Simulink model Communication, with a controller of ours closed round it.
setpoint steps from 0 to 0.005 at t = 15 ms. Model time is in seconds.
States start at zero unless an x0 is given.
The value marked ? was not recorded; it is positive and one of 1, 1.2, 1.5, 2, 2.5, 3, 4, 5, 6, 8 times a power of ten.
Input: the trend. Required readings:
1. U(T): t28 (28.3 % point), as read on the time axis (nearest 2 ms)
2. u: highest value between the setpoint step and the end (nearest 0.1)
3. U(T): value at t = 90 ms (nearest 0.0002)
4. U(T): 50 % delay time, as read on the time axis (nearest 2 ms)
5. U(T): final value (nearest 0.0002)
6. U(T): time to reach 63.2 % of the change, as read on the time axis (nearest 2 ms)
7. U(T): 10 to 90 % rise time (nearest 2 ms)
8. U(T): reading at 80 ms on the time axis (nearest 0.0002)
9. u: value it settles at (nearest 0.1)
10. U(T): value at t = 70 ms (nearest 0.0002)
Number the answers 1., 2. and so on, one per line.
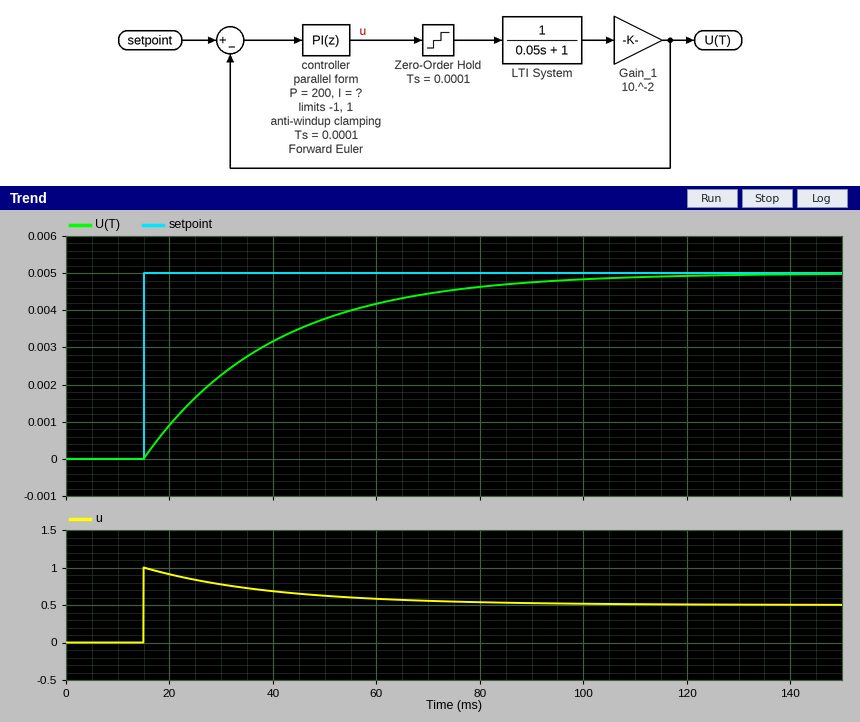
1. 24 ms
2. 1.0
3. 0.0048
4. 32 ms
5. 0.0050
6. 40 ms
7. 54 ms
8. 0.0046
9. 0.5
10. 0.0044
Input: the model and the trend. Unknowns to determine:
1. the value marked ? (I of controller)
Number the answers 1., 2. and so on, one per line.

1. 4000
